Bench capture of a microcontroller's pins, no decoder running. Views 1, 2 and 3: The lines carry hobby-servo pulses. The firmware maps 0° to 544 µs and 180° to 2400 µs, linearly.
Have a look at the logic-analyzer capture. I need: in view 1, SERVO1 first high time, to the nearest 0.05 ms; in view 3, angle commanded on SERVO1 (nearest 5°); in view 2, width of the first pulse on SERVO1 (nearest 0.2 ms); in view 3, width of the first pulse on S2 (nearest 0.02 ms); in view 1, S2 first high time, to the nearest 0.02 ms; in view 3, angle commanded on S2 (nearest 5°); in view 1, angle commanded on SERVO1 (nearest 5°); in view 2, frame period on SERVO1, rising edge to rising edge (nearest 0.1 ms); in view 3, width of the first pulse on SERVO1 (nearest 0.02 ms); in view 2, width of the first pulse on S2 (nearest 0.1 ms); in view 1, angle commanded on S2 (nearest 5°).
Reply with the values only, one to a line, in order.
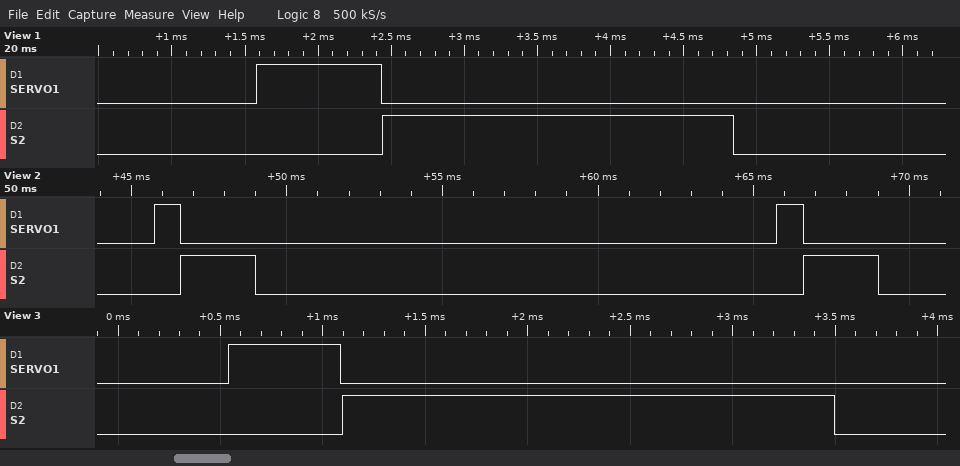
0.85 ms
0°
0.8 ms
2.40 ms
2.40 ms
180°
30°
20.0 ms
0.54 ms
2.4 ms
180°
